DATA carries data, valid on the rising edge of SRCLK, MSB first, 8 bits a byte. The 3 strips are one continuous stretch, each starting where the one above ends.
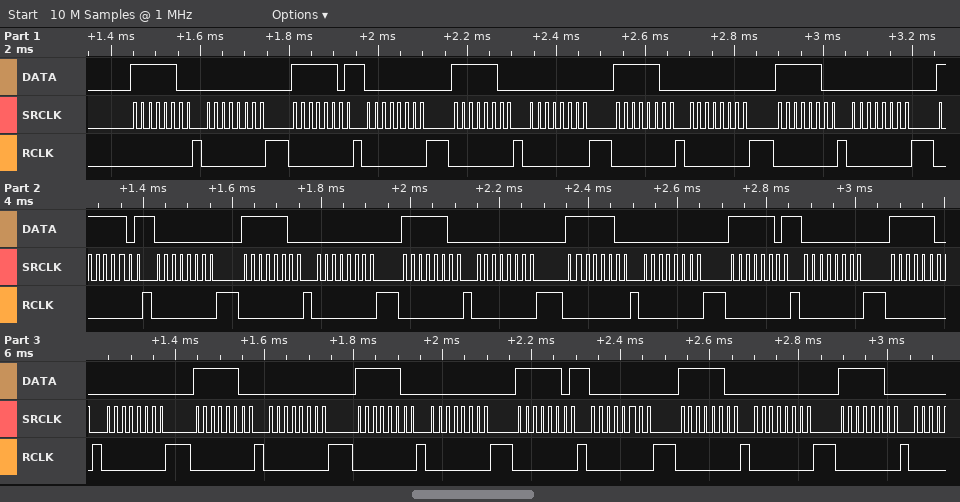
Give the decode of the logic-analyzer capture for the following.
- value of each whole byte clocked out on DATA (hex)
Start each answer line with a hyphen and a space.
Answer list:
- FC 00 FD 00 FC 00 FC 00 FC 00 FD 00 FC 00 FC 00 FC 00 FD 00 FC 00 FC 00 FC 00 FD 00 FC 00 FC
